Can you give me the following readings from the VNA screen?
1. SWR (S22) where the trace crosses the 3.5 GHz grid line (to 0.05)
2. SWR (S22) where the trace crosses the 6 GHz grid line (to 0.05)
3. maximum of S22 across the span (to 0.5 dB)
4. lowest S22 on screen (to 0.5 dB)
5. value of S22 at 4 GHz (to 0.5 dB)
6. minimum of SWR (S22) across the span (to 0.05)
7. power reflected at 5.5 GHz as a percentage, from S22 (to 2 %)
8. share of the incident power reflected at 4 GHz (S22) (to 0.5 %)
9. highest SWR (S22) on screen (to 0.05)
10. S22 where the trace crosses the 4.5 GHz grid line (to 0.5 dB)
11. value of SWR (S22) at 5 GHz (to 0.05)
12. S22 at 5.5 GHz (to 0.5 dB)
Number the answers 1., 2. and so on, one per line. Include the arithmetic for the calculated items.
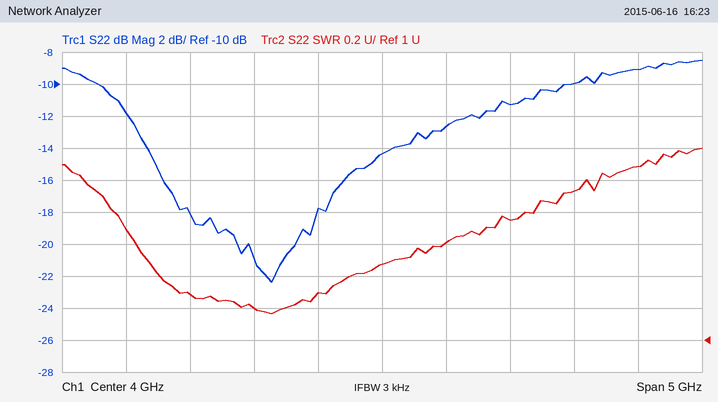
1. 1.30
2. 2.10
3. -8.5 dB
4. -22.5 dB
5. -14.5 dB
6. 1.15
7. 10^(-10/10) ≈ 10 %
8. 10^(-14.5/10) ≈ 3.5 %
9. 2.20
10. -12.5 dB
11. 1.75
12. -10.0 dB
